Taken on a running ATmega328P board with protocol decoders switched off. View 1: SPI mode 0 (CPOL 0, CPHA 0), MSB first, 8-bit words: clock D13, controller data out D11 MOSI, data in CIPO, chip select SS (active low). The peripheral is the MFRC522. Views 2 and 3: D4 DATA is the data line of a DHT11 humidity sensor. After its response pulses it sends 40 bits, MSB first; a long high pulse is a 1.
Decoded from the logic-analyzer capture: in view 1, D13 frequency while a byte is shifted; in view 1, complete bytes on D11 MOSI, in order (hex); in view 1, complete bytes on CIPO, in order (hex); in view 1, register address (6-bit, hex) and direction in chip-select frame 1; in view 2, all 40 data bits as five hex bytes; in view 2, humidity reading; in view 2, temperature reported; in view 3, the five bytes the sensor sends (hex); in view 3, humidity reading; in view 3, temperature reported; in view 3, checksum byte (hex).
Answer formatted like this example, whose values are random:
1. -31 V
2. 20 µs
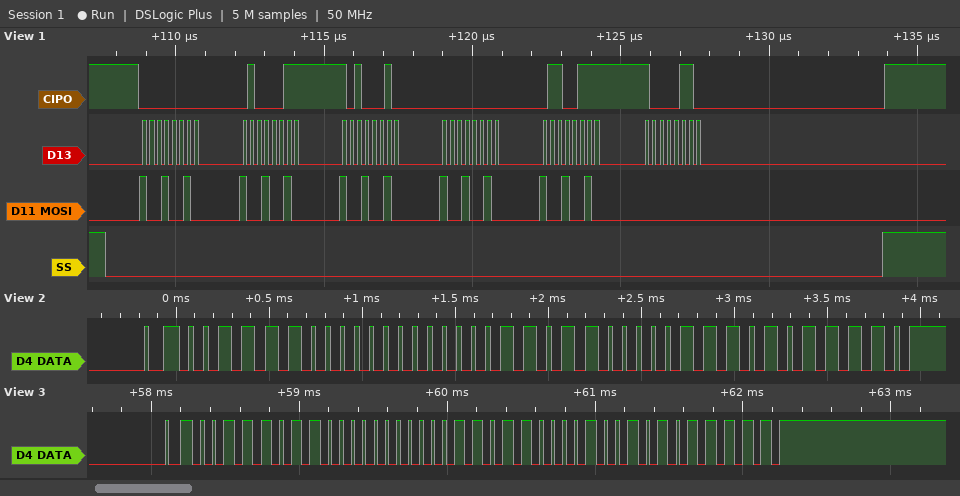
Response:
1. 4 MHz
2. 92 92 92 92 92 00
3. 00 43 A2 00 67 86
4. 0x09 read
5. 3C 00 1B 07 5E
6. 60 %
7. 27.7 °C
8. 3B 00 1B 09 5F
9. 59 %
10. 27.9 °C
11. 0x5F
